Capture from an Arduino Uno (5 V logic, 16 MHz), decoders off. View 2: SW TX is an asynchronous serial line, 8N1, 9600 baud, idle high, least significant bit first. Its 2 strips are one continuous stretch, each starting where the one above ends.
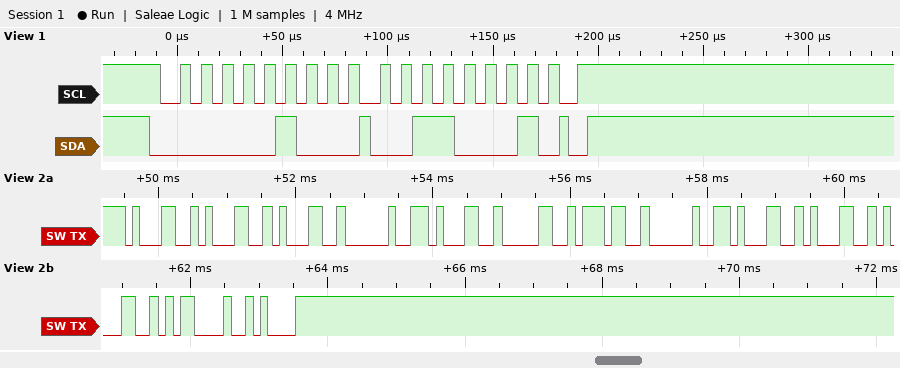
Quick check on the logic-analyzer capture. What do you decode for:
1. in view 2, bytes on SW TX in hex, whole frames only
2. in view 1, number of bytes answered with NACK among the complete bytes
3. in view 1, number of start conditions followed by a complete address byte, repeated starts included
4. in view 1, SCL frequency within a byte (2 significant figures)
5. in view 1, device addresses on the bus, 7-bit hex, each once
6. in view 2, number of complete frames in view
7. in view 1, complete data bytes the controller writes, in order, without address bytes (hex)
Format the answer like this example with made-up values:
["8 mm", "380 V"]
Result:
["0x31 0x31 0x31 0x20 0x31 0x30 0x37 0x20 0x31 0x31 0x31 0x0D 0x0A", "0", "1", "100 kHz", "0x02", "13", "31"]
